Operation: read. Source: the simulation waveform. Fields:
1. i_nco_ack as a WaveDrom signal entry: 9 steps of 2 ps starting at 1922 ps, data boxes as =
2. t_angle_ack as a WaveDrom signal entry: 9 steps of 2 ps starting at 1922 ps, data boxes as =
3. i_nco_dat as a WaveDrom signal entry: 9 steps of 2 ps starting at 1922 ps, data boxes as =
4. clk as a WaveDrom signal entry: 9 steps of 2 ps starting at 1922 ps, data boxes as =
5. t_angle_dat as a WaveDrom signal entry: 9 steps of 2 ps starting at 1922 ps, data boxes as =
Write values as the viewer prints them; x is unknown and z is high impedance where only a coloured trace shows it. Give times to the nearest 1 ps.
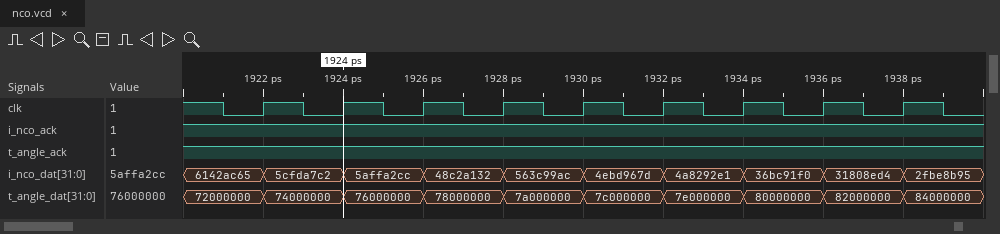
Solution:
{name: 'i_nco_ack', wave: '1........'}
{name: 't_angle_ack', wave: '1........'}
{name: 'i_nco_dat', wave: '=========', data: '5cfda7c2 5affa2cc 48c2a132 563c99ac 4ebd967d 4a8292e1 36bc91f0 31808ed4 2fbe8b95'}
{name: 'clk', wave: 'p........'}
{name: 't_angle_dat', wave: '=========', data: '74000000 76000000 78000000 7a000000 7c000000 7e000000 80000000 82000000 84000000'}
